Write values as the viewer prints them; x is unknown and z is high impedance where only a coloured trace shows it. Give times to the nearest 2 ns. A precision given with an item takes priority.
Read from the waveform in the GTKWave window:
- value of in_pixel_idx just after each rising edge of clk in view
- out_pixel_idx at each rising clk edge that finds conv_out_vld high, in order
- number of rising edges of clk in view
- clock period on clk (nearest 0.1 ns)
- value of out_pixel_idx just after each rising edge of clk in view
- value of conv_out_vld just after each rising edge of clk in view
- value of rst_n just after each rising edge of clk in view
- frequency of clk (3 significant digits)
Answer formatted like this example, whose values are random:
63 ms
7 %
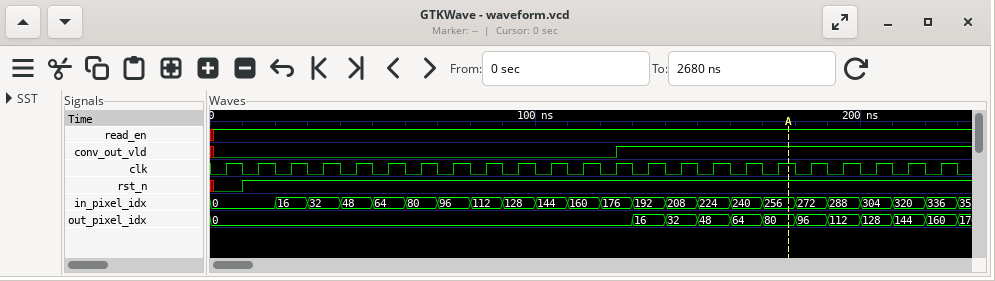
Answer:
0, 0, 16, 32, 48, 64, 80, 96, 112, 128, 144, 160, 176, 192, 208, 224, 240, 256, 272, 288, 304, 320, 336
16, 32, 48, 64, 80, 96, 112, 128, 144, 160
23
10 ns
0, 0, 0, 0, 0, 0, 0, 0, 0, 0, 0, 0, 0, 16, 32, 48, 64, 80, 96, 112, 128, 144, 160
0 0 0 0 0 0 0 0 0 0 0 0 1 1 1 1 1 1 1 1 1 1 1
0 1 1 1 1 1 1 1 1 1 1 1 1 1 1 1 1 1 1 1 1 1 1
100 MHz
